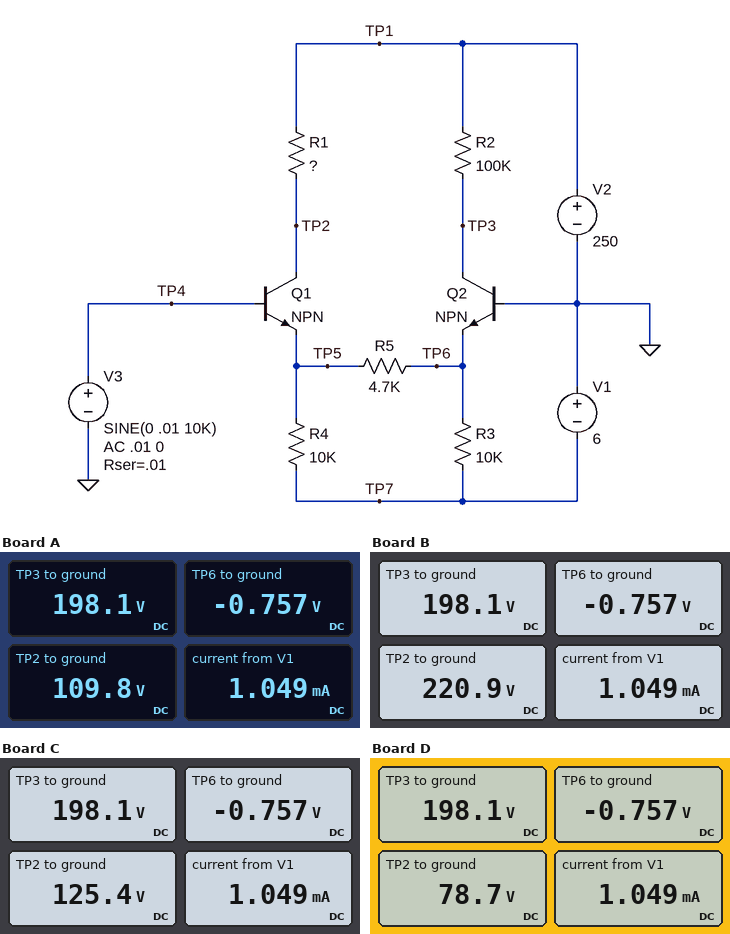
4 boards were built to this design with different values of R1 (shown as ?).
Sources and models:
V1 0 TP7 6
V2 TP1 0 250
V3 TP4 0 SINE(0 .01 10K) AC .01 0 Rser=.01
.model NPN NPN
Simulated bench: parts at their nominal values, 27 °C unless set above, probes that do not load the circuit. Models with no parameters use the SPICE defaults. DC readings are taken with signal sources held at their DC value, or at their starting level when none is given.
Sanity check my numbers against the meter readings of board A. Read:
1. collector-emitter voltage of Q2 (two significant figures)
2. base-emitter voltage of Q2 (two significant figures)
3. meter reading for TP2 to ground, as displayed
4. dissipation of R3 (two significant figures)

200 V
760 mV
109.8 V
2.7 mW
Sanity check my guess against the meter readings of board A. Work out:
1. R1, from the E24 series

270 kΩ
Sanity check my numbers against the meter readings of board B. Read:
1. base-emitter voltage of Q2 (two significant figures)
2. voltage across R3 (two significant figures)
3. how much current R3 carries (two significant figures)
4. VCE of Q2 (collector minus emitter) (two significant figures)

760 mV
5.2 V
520 µA
200 V
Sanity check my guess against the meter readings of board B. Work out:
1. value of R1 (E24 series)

56 kΩ
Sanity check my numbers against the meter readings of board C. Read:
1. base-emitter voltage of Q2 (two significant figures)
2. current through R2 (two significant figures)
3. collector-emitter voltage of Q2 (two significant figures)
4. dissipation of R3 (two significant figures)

760 mV
520 µA
200 V
2.7 mW
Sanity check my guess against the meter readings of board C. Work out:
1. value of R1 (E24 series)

240 kΩ
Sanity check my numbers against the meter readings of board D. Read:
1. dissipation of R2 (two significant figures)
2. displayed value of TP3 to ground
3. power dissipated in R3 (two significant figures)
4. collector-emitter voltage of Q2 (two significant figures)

27 mW
198.1 V
2.7 mW
200 V
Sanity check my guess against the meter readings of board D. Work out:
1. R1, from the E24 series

330 kΩ
